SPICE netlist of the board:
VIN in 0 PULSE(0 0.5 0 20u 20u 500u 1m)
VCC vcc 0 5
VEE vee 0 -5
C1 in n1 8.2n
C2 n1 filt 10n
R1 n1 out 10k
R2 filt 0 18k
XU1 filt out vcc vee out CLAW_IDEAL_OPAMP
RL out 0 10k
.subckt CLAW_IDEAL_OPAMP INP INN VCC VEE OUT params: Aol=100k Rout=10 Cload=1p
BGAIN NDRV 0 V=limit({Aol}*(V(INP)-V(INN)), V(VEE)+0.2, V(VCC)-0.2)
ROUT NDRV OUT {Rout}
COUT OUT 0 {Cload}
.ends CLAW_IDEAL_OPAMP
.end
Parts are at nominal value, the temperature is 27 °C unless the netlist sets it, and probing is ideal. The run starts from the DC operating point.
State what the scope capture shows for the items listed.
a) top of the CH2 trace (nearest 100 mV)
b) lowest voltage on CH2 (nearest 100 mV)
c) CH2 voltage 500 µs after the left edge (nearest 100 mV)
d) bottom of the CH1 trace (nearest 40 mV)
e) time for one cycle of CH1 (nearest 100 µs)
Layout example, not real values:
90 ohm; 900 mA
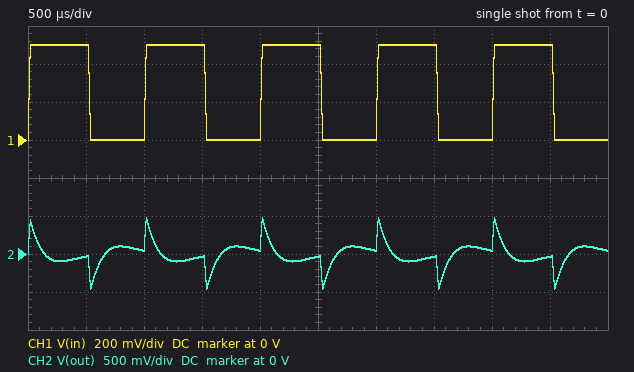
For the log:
500 mV; -500 mV; 0 V; 0 V; 1.0 ms
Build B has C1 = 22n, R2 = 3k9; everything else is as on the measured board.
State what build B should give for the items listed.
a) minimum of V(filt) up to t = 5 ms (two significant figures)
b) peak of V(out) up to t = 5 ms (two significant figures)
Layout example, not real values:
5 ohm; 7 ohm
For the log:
-360 mV; 360 mV
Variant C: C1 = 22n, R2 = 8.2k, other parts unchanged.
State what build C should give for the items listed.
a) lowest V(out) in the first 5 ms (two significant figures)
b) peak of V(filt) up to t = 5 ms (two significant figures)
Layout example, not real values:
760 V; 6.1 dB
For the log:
-440 mV; 440 mV
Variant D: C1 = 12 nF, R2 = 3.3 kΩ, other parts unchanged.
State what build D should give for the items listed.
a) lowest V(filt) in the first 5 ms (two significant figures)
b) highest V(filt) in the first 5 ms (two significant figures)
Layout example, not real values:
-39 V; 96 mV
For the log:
-300 mV; 300 mV
